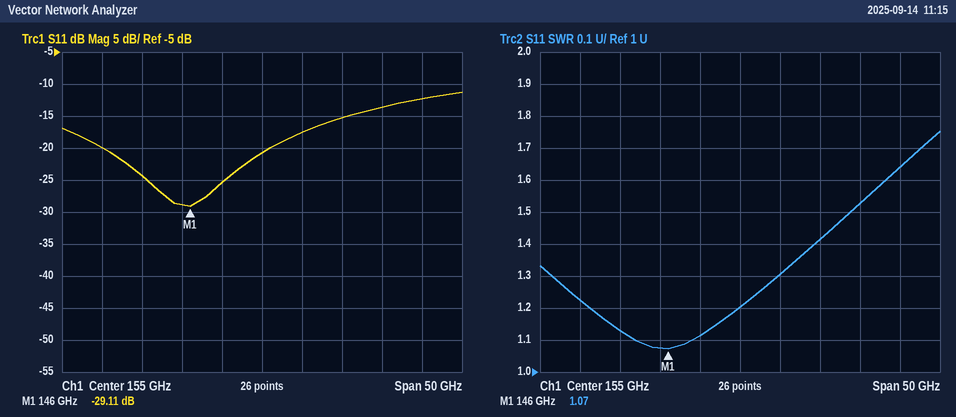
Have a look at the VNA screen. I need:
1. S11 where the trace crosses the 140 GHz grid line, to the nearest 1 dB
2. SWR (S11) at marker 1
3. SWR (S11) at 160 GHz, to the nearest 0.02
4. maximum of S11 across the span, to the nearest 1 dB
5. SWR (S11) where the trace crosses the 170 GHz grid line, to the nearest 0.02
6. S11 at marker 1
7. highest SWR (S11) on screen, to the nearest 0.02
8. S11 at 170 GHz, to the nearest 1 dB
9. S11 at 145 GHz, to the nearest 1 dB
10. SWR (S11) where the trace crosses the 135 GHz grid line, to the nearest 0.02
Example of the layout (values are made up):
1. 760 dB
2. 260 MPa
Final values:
1. -24 dB
2. 1.07
3. 1.30
4. -11 dB
5. 1.52
6. -29.11 dB
7. 1.76
8. -14 dB
9. -29 dB
10. 1.22
